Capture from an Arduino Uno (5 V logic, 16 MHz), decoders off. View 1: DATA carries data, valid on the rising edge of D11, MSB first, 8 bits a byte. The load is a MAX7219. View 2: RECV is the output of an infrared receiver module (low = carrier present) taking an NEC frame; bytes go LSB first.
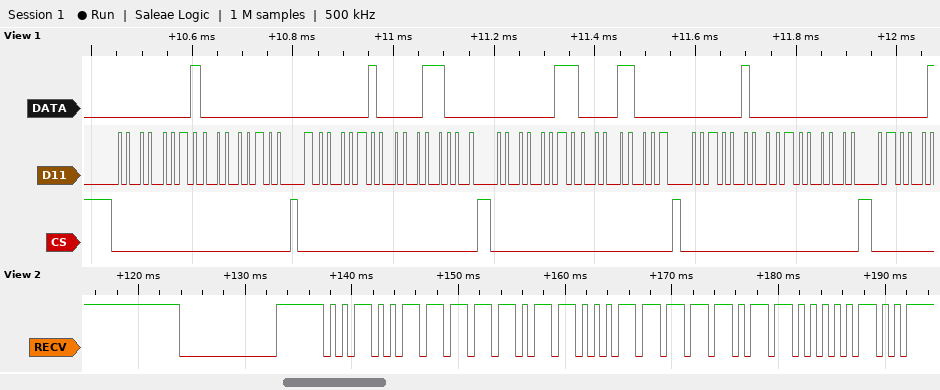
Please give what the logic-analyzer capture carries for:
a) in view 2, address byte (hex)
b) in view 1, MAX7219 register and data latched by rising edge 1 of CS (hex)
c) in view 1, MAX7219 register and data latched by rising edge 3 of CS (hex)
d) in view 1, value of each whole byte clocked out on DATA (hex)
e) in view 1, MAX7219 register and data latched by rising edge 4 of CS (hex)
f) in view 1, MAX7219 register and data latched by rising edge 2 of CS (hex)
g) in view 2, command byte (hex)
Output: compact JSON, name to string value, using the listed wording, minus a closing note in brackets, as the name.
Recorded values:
{"in view 2, address byte": "0xE4", "in view 1, MAX7219 register and data latched by rising edge 1 of CS": "register 0x1, data 0x00", "in view 1, MAX7219 register and data latched by rising edge 3 of CS": "register 0x3, data 0x18", "in view 1, value of each whole byte clocked out on DATA": "0x01 0x00 0x02 0x18 0x03 0x18 0x04 0x00", "in view 1, MAX7219 register and data latched by rising edge 4 of CS": "register 0x4, data 0x00", "in view 1, MAX7219 register and data latched by rising edge 2 of CS": "register 0x2, data 0x18", "in view 2, command byte": "0xDF"}
